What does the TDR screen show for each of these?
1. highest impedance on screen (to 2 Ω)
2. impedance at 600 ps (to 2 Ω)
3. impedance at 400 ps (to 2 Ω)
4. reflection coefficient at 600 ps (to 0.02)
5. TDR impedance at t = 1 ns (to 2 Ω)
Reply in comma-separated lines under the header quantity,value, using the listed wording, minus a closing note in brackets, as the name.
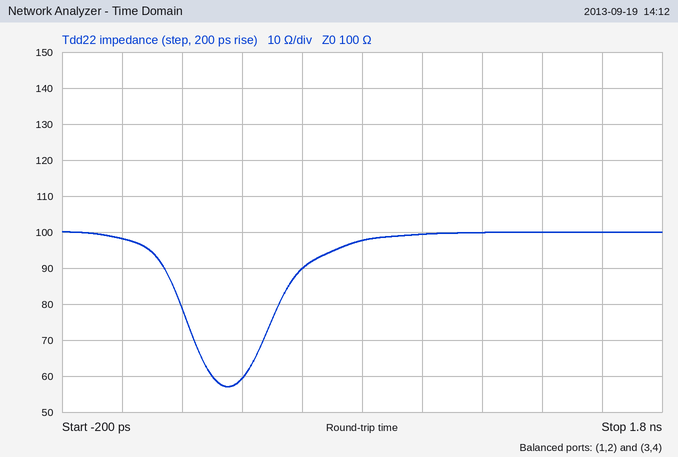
quantity,value
highest impedance on screen,100 Ω
impedance at 600 ps,90 Ω
impedance at 400 ps,60 Ω
reflection coefficient at 600 ps,-0.06
TDR impedance at t = 1 ns,100 Ω
